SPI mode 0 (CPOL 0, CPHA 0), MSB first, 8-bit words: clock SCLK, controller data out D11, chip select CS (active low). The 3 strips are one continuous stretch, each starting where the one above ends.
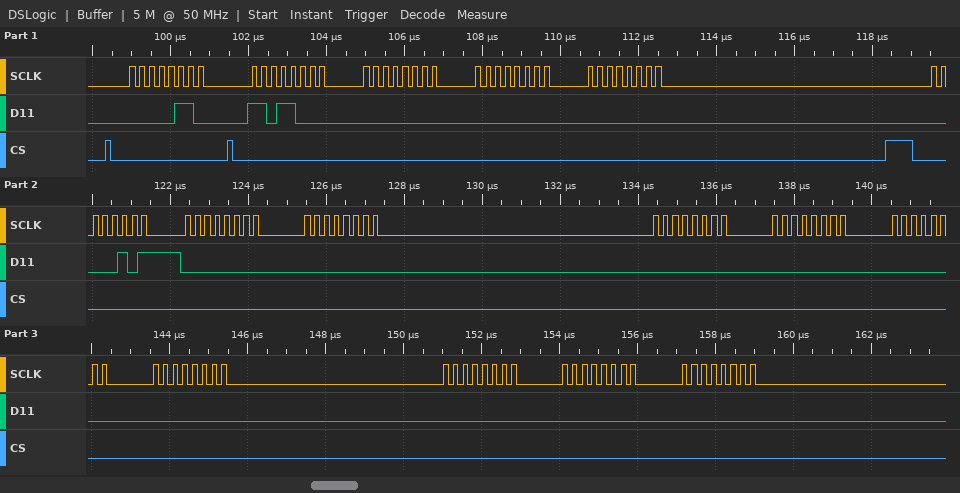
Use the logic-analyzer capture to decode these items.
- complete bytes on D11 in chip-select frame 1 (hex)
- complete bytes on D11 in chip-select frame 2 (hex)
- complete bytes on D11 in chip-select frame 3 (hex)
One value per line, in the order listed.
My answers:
06
D8 00 00 00
05 00 00 00 00 00 00 00 00 00
